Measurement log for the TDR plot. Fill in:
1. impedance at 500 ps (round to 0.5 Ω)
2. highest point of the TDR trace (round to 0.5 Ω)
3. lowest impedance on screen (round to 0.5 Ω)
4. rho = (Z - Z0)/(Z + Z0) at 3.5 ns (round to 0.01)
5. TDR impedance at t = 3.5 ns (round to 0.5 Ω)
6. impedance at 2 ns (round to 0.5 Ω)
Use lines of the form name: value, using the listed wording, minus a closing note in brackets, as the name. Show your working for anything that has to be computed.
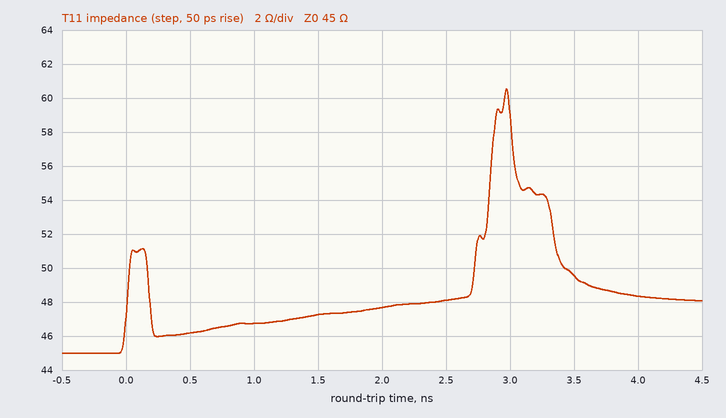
impedance at 500 ps: 46.0 Ω
highest point of the TDR trace: 60.5 Ω
lowest impedance on screen: 45.0 Ω
rho = (Z - Z0)/(Z + Z0) at 3.5 ns: (49.5 − 45)/(49.5 + 45) ≈ +0.05
TDR impedance at t = 3.5 ns: 49.5 Ω
impedance at 2 ns: 47.5 Ω
